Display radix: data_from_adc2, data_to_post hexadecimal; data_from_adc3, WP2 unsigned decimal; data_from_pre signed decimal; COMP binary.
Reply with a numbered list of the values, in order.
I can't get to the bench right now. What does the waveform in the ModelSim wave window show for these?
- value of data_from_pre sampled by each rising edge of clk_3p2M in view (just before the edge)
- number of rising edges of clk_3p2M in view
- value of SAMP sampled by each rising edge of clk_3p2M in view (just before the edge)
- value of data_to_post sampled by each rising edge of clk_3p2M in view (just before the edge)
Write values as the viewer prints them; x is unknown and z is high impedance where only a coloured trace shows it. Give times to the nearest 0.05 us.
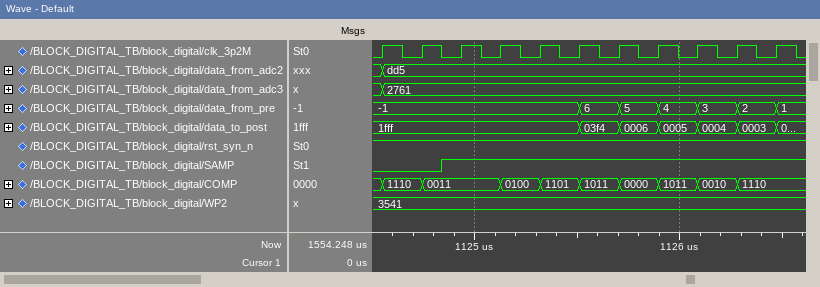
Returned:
1. -1, -1, -1, -1, -1, -1, 6, 5, 4, 3, 2
2. 11
3. 0 0 1 1 1 1 1 1 1 1 1
4. 1fff, 1fff, 1fff, 1fff, 1fff, 1fff, 03f4, 0006, 0005, 0004, 0003
